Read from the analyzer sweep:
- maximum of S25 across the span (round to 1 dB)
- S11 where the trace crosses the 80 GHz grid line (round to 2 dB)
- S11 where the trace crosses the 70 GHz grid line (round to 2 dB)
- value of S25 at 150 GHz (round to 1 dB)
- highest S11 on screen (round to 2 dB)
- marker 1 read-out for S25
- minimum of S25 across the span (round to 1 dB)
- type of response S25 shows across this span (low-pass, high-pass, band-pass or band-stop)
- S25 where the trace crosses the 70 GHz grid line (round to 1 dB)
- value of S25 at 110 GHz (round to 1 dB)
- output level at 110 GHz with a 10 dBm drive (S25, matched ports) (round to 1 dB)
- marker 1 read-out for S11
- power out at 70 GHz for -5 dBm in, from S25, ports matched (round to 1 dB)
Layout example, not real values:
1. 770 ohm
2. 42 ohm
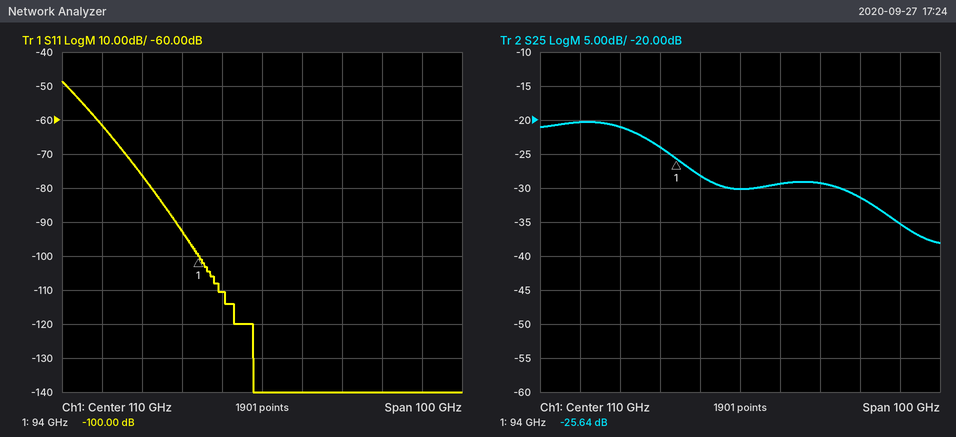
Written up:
1. -20 dB
2. -76 dB
3. -62 dB
4. -35 dB
5. -48 dB
6. -25.64 dB
7. -38 dB
8. low-pass
9. -20 dB
10. -30 dB
11. -20 dBm
12. -100.00 dB
13. -25 dBm
